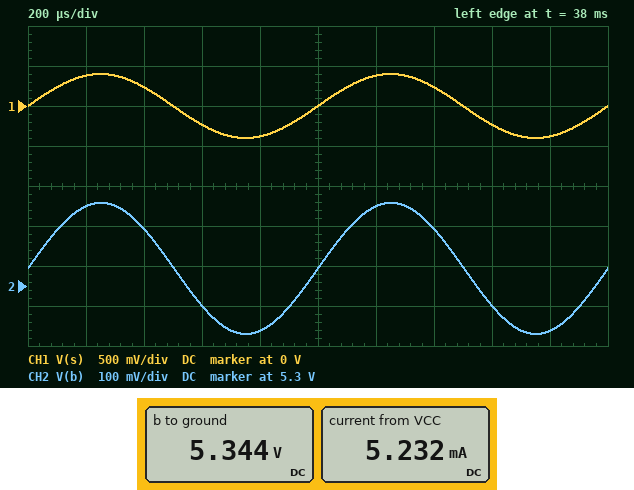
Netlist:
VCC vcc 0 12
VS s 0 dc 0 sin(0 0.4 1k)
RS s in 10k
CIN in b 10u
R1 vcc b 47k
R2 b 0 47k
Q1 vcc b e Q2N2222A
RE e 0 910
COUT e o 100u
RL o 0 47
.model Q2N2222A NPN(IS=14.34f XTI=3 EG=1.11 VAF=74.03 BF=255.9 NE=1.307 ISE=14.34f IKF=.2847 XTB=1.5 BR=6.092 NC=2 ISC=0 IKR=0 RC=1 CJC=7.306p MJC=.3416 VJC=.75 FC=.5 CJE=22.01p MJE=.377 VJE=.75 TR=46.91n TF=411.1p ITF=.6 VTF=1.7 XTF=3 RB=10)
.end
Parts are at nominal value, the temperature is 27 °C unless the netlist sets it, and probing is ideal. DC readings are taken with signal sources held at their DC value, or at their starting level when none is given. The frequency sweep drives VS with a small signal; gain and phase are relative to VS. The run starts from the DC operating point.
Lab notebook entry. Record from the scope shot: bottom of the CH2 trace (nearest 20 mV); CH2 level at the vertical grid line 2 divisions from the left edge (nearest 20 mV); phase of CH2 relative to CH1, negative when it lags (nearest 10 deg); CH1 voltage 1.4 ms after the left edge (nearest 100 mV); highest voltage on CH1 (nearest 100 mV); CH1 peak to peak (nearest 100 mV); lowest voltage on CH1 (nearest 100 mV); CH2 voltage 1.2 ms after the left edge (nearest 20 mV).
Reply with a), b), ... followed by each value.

a) 5.18 V
b) 5.44 V
c) 0 deg
d) 200 mV
e) 400 mV
f) 800 mV
g) -400 mV
h) 5.50 V
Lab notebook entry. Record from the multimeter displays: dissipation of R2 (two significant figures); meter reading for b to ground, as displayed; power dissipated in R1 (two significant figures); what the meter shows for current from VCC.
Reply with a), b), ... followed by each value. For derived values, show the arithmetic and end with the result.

a) (5.344 V)^2 / 47 kΩ = 610 µW
b) 5.344 V
c) (12 V - 5.344 V)^2 / 47 kΩ = 940 µW
d) 5.232 mA
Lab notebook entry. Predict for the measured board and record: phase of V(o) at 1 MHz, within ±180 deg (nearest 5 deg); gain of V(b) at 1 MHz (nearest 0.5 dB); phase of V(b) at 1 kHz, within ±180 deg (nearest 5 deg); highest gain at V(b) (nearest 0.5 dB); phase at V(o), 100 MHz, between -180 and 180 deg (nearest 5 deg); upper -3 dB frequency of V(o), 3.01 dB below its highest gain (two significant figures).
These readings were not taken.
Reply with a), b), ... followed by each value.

a) -20 deg
b) -8.5 dB
c) 0 deg
d) -4.0 dB
e) -70 deg
f) 2.5 MHz
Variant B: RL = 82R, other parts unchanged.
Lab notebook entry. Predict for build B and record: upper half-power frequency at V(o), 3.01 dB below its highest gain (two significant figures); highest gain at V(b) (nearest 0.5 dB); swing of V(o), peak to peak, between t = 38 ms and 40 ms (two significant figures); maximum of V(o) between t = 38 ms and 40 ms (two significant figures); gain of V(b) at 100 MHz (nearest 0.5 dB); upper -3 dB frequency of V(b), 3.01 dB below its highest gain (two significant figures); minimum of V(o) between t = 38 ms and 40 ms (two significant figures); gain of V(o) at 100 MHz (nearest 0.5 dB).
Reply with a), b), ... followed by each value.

a) 3.0 MHz
b) -4.0 dB
c) 360 mV
d) 180 mV
e) -36.0 dB
f) 1.1 MHz
g) -180 mV
h) -37.0 dB
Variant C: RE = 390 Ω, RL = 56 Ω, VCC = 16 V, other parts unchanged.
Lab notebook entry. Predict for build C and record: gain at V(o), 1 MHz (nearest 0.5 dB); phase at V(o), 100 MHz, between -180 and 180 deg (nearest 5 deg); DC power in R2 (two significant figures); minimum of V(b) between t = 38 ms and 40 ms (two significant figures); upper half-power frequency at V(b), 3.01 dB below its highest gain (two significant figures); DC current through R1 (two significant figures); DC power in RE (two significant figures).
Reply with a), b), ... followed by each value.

a) -8.5 dB
b) -75 deg
c) 850 µW
d) 6.1 V
e) 69 Hz
f) 210 µA
g) 80 mW
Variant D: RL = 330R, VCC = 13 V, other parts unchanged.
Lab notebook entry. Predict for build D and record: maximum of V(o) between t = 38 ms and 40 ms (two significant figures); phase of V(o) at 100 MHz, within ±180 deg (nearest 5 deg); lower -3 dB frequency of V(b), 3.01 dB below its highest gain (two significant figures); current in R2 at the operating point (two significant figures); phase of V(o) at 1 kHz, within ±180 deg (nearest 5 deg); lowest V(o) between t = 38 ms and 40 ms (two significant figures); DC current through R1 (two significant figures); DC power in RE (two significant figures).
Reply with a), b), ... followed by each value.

a) 240 mV
b) -80 deg
c) 470 mHz
d) 120 µA
e) 0 deg
f) -240 mV
g) 150 µA
h) 29 mW
